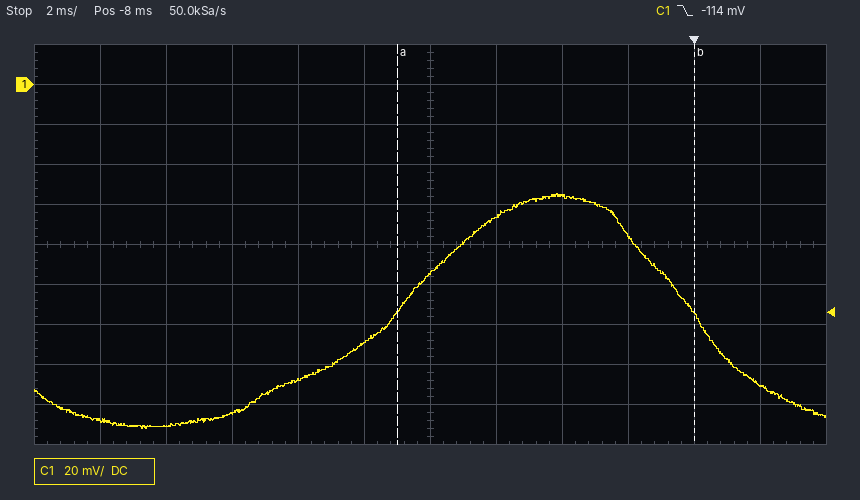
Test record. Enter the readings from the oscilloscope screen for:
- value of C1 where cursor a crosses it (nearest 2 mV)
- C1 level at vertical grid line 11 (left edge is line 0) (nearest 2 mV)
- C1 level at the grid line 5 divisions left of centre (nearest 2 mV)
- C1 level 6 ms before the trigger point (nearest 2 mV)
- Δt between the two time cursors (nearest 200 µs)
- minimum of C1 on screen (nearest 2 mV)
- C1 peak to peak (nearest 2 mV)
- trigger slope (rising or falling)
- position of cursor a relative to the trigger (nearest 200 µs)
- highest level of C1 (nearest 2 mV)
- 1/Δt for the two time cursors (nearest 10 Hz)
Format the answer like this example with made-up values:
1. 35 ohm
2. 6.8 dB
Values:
1. -114 mV
2. -150 mV
3. -168 mV
4. -66 mV
5. 9.0 ms
6. -172 mV
7. 118 mV
8. falling
9. -9.0 ms
10. -54 mV
11. 110 Hz
